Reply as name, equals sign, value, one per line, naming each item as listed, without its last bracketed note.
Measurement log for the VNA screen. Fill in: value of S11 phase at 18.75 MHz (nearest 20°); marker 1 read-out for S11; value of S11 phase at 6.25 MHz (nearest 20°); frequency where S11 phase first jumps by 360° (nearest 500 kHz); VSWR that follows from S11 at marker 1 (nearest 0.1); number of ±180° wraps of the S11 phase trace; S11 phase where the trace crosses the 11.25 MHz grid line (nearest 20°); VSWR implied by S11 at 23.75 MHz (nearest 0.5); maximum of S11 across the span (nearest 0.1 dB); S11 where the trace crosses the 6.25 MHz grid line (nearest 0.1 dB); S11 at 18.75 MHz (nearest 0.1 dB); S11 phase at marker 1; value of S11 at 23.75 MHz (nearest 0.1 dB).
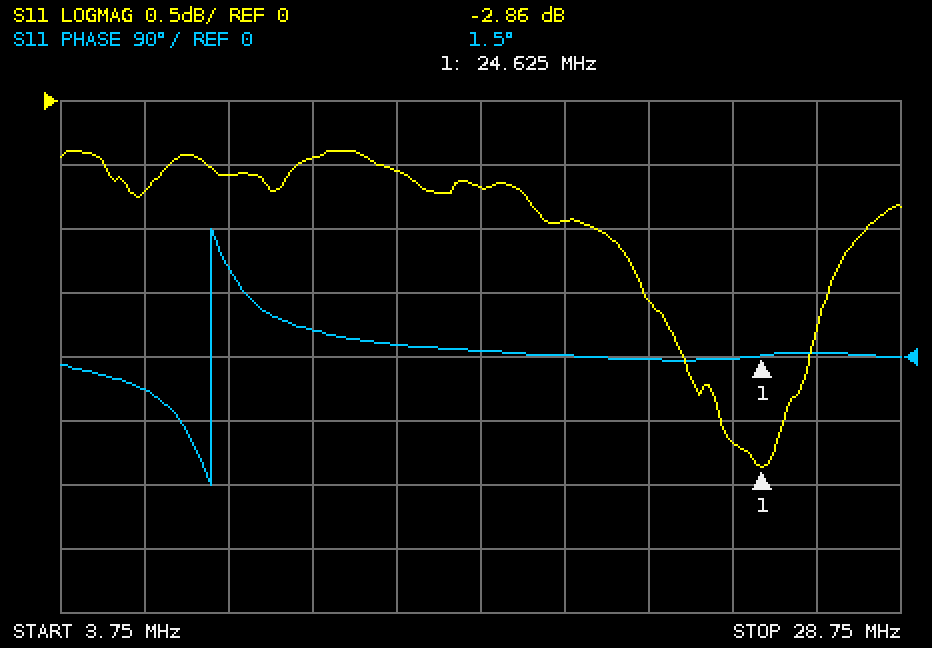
value of S11 phase at 18.75 MHz = 0°
marker 1 read-out for S11 = -2.86 dB
value of S11 phase at 6.25 MHz = -40°
frequency where S11 phase first jumps by 360° = 8.0 MHz
VSWR that follows from S11 at marker 1 = 6.1
number of ±180° wraps of the S11 phase trace = 1
S11 phase where the trace crosses the 11.25 MHz grid line = 40°
VSWR implied by S11 at 23.75 MHz = 6.5
maximum of S11 across the span = -0.4 dB
S11 where the trace crosses the 6.25 MHz grid line = -0.7 dB
S11 at 18.75 MHz = -0.9 dB
S11 phase at marker 1 = 1.5°
value of S11 at 23.75 MHz = -2.7 dB
